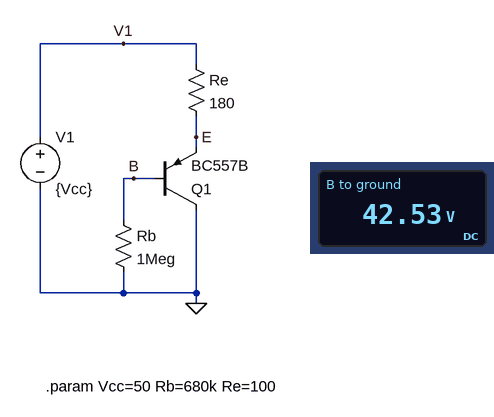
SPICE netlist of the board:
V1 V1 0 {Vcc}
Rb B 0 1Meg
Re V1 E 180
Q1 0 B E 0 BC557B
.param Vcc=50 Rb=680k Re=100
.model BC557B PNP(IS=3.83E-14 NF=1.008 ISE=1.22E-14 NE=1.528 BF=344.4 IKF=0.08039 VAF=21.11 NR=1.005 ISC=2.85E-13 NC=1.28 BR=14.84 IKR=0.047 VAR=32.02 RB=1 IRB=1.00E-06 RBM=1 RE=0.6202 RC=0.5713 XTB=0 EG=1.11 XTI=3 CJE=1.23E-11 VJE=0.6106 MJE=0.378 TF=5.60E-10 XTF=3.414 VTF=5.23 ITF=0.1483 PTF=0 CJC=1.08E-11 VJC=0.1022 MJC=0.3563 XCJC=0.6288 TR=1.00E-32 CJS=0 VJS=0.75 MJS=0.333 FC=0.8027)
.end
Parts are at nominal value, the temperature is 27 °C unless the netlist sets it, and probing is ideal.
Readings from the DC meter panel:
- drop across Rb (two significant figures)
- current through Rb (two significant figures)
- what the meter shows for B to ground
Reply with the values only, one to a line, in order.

43 V
43 µA
42.53 V
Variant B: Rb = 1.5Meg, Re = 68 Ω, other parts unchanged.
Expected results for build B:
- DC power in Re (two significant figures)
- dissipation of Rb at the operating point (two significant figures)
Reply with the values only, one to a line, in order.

64 mW
1.5 mW
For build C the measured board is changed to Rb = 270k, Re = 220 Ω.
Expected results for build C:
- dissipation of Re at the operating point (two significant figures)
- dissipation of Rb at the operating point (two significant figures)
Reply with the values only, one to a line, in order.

1.3 W
3.9 mW
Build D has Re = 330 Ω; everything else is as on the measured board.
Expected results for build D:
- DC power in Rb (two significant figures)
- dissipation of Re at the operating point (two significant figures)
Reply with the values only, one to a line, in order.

1.5 mW
340 mW
